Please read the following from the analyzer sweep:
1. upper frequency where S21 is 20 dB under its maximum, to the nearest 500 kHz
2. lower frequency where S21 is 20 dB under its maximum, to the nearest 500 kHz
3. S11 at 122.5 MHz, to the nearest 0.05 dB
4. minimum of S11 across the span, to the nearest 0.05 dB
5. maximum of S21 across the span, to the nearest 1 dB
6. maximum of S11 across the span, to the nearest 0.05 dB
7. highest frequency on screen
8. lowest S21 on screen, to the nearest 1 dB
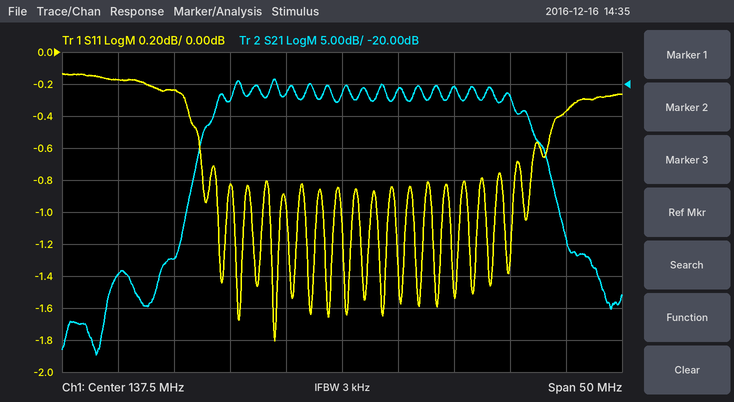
157.0 MHz
123.5 MHz
-0.25 dB
-1.80 dB
-19 dB
-0.15 dB
162.5 MHz
-62 dB
